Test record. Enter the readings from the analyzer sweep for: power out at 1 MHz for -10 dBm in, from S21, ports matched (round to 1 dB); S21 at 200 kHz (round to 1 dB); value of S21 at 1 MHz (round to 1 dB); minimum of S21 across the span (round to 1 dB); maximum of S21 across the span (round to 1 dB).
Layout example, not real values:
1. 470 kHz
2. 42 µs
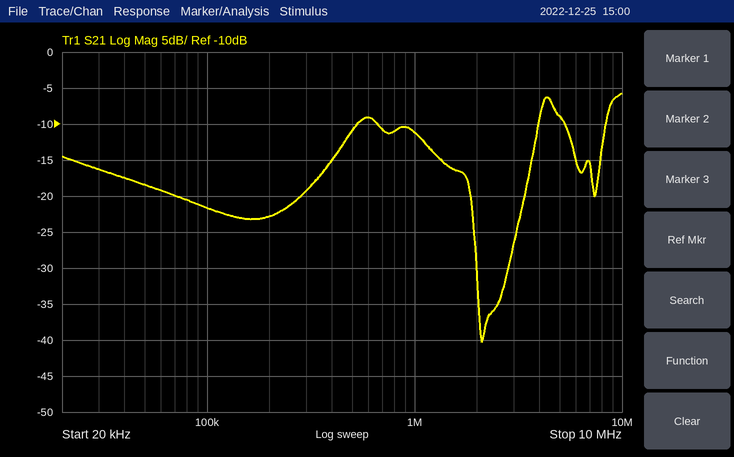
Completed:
1. -21 dBm
2. -23 dB
3. -11 dB
4. -40 dB
5. -6 dB
